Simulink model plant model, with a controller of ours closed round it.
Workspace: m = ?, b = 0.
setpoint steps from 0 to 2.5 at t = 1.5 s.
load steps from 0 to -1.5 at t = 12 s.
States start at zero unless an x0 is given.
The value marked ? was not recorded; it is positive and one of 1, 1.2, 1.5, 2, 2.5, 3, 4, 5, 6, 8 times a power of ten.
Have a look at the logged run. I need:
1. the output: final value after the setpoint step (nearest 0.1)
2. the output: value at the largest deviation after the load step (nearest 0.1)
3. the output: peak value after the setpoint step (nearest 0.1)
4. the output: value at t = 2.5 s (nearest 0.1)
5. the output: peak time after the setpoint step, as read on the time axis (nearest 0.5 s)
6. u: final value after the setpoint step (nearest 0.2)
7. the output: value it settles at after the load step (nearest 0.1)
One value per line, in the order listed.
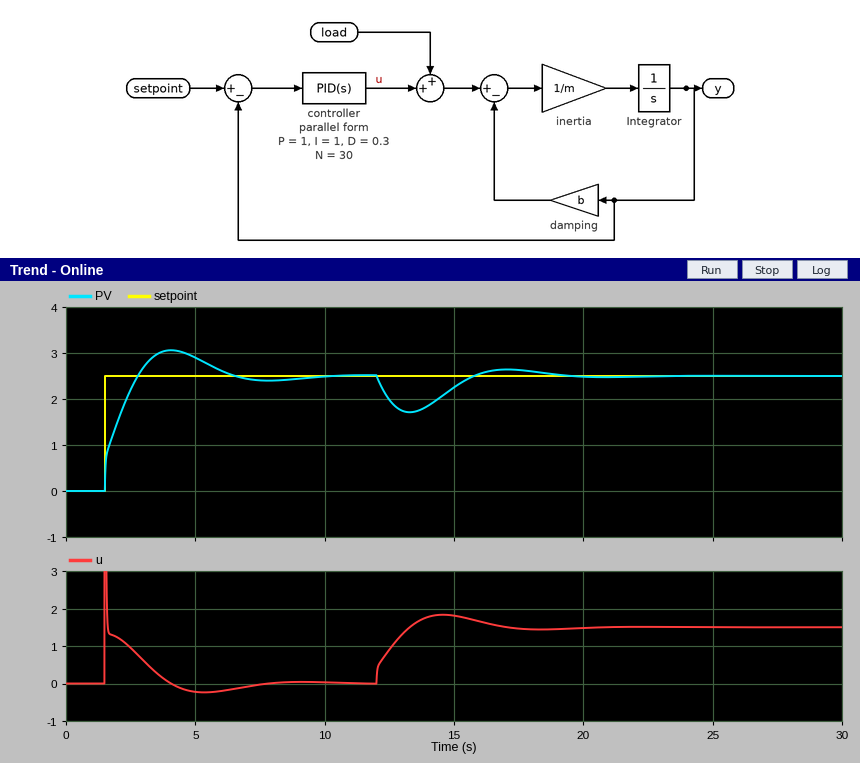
2.5
1.7
3.1
2.2
4.0 s
0.0
2.5
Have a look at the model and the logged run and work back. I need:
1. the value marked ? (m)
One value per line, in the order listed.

0.8
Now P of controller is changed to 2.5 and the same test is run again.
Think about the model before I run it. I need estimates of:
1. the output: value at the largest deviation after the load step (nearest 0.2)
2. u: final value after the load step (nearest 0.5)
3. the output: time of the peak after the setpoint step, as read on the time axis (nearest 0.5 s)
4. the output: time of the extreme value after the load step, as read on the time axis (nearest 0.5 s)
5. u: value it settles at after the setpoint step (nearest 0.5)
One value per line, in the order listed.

2.0
1.5
3.5 s
13.0 s
0.0
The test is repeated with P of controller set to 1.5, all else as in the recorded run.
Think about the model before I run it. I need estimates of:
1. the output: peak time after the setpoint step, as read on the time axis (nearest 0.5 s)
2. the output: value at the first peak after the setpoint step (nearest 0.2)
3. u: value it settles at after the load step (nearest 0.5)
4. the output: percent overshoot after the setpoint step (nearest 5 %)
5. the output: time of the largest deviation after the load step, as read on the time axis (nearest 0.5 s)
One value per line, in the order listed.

4.0 s
2.8
1.5
15 %
13.0 s
